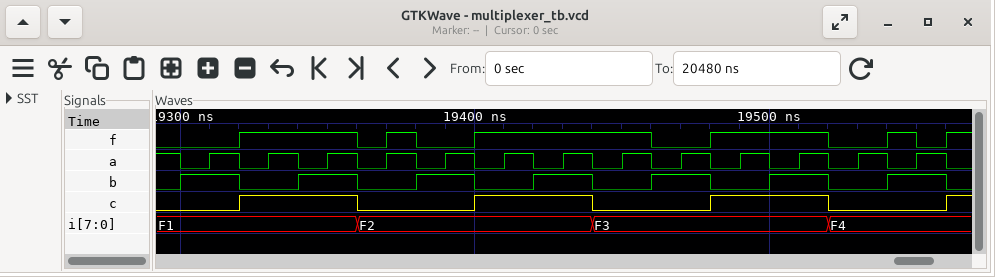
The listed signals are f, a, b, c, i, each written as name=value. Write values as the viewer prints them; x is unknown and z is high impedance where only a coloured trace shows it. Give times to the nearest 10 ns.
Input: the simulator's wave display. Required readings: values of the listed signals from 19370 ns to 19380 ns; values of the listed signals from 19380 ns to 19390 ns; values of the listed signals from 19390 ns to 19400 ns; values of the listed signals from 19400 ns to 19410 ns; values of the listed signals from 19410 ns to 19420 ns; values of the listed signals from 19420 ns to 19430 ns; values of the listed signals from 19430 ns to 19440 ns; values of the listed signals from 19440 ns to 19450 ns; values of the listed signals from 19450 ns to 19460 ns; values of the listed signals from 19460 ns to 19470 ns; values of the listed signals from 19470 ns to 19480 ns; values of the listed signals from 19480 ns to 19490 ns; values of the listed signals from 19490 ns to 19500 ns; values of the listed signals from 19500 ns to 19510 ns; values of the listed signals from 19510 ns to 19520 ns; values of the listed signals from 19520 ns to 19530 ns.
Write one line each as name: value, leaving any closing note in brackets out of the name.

values of the listed signals from 19370 ns to 19380 ns: f=1, a=1, b=0, c=0, i=F2
values of the listed signals from 19380 ns to 19390 ns: f=0, a=0, b=1, c=0, i=F2
values of the listed signals from 19390 ns to 19400 ns: f=0, a=1, b=1, c=0, i=F2
values of the listed signals from 19400 ns to 19410 ns: f=1, a=0, b=0, c=1, i=F2
values of the listed signals from 19410 ns to 19420 ns: f=1, a=1, b=0, c=1, i=F2
values of the listed signals from 19420 ns to 19430 ns: f=1, a=0, b=1, c=1, i=F2
values of the listed signals from 19430 ns to 19440 ns: f=1, a=1, b=1, c=1, i=F2
values of the listed signals from 19440 ns to 19450 ns: f=1, a=0, b=0, c=0, i=F3
values of the listed signals from 19450 ns to 19460 ns: f=1, a=1, b=0, c=0, i=F3
values of the listed signals from 19460 ns to 19470 ns: f=0, a=0, b=1, c=0, i=F3
values of the listed signals from 19470 ns to 19480 ns: f=0, a=1, b=1, c=0, i=F3
values of the listed signals from 19480 ns to 19490 ns: f=1, a=0, b=0, c=1, i=F3
values of the listed signals from 19490 ns to 19500 ns: f=1, a=1, b=0, c=1, i=F3
values of the listed signals from 19500 ns to 19510 ns: f=1, a=0, b=1, c=1, i=F3
values of the listed signals from 19510 ns to 19520 ns: f=1, a=1, b=1, c=1, i=F3
values of the listed signals from 19520 ns to 19530 ns: f=0, a=0, b=0, c=0, i=F4
